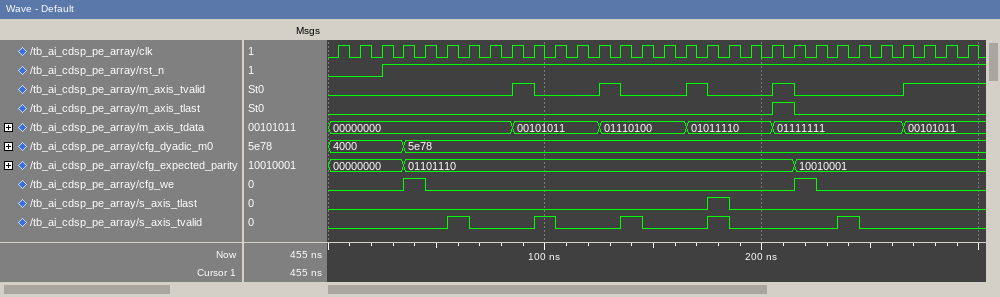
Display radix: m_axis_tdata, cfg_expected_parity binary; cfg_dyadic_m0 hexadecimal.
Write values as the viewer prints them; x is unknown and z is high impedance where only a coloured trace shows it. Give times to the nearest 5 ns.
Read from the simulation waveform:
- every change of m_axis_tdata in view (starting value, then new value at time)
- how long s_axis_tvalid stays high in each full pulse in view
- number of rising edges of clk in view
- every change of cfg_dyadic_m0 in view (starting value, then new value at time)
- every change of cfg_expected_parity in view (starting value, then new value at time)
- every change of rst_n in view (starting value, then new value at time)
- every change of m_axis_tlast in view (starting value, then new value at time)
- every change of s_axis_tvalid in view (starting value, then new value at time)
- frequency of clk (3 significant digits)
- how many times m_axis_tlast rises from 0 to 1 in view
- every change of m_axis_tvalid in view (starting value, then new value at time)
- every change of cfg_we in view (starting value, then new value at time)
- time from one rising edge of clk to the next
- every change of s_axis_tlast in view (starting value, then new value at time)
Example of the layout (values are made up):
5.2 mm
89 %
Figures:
00000000, 00101011 at 85 ns, 01110100 at 125 ns, 01011110 at 165 ns, 01111111 at 205 ns, 00101011 at 265 ns
10 ns, 10 ns, 10 ns, 10 ns, 10 ns
30
4000, 5e78 at 35 ns
00000000, 01101110 at 35 ns, 10010001 at 215 ns
0, 1 at 25 ns
0, 1 at 205 ns, 0 at 215 ns
0, 1 at 55 ns, 0 at 65 ns, 1 at 95 ns, 0 at 105 ns, 1 at 135 ns, 0 at 145 ns, 1 at 175 ns, 0 at 185 ns, 1 at 235 ns, 0 at 245 ns
100 MHz
1
0, 1 at 85 ns, 0 at 95 ns, 1 at 125 ns, 0 at 135 ns, 1 at 165 ns, 0 at 175 ns, 1 at 205 ns, 0 at 215 ns, 1 at 265 ns
0, 1 at 35 ns, 0 at 45 ns, 1 at 215 ns, 0 at 225 ns
10 ns
0, 1 at 175 ns, 0 at 185 ns
